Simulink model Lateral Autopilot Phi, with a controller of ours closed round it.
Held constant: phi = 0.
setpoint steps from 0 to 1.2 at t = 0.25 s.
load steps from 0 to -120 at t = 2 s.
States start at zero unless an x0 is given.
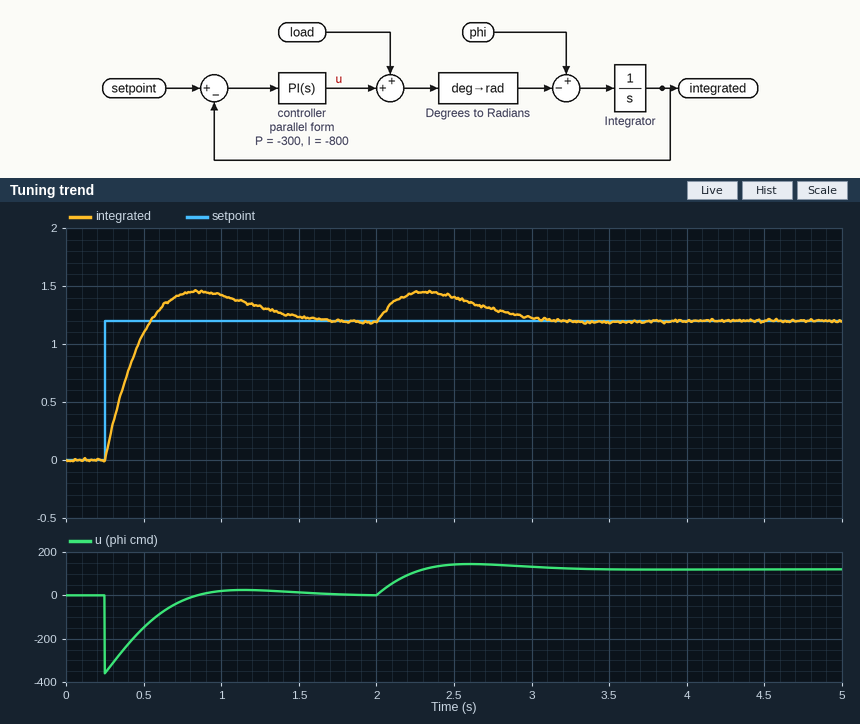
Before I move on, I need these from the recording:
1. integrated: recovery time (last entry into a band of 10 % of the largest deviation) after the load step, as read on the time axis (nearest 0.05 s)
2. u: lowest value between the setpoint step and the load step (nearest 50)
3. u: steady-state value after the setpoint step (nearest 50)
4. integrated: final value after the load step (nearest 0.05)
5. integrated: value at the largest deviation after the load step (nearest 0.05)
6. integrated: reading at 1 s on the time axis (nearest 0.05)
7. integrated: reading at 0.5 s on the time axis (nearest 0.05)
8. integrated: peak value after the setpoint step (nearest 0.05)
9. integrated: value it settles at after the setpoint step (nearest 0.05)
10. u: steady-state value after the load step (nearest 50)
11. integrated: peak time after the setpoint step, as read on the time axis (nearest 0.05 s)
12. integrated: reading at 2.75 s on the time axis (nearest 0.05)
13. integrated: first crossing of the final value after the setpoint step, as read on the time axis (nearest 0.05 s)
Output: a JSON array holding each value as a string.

["3.00 s", "-350", "0", "1.20", "1.45", "1.40", "1.10", "1.45", "1.20", "100", "0.85 s", "1.30", "0.55 s"]
